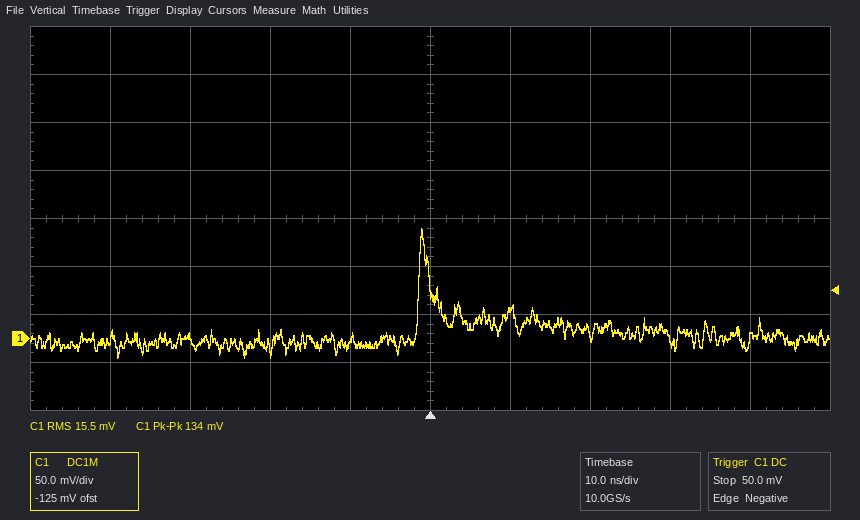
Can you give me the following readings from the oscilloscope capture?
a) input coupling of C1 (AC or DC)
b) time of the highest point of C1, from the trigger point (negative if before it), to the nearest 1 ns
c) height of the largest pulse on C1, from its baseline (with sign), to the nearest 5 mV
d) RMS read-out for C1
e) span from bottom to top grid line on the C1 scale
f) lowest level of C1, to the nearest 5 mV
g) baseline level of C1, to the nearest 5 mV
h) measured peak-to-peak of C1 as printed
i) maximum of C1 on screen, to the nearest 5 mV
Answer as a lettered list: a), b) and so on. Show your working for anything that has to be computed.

a) DC
b) -1 ns
c) 115 mV − (0 mV) = +115 mV
d) 15.5 mV
e) 400 mV
f) -20 mV
g) 0 mV
h) 134 mV
i) 115 mV
